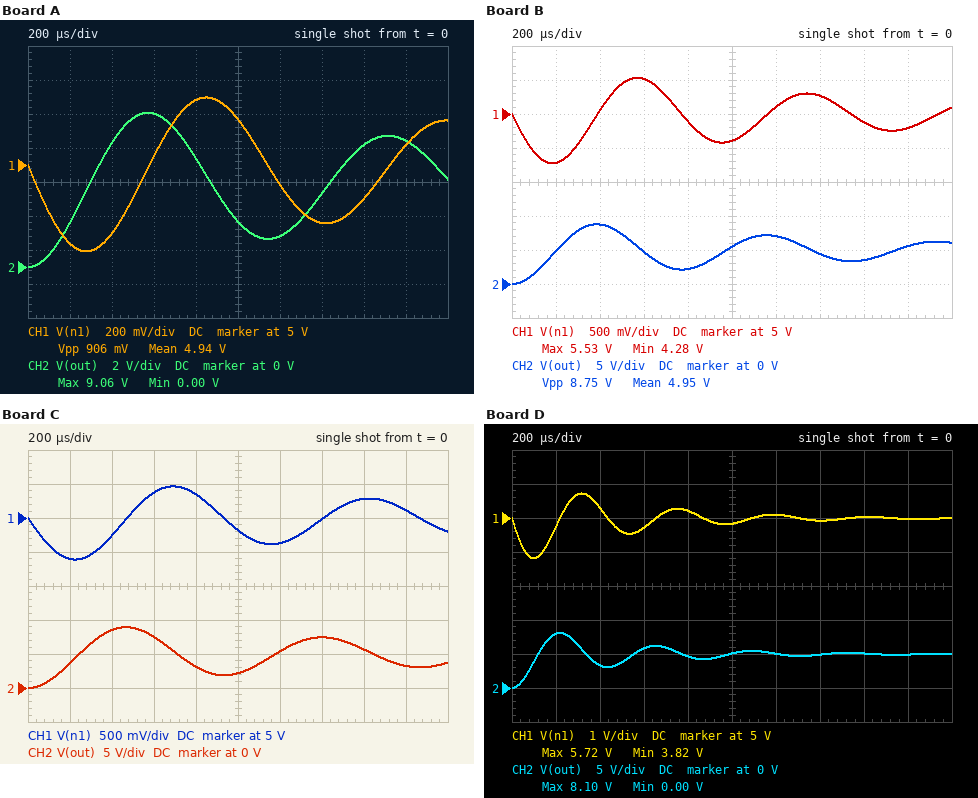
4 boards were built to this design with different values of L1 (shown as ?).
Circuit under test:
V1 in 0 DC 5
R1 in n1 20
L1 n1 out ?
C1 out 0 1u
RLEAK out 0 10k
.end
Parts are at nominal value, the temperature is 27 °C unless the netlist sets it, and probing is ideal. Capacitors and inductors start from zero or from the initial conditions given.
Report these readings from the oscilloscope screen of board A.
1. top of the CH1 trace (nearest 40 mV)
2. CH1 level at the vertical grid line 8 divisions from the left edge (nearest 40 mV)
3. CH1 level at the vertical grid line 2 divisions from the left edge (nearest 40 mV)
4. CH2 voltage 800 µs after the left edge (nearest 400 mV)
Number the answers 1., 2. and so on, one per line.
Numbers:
1. 5.40 V
2. 4.80 V
3. 4.60 V
4. 6.4 V
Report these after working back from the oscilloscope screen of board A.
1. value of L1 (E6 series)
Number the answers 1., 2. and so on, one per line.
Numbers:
1. 33 mH
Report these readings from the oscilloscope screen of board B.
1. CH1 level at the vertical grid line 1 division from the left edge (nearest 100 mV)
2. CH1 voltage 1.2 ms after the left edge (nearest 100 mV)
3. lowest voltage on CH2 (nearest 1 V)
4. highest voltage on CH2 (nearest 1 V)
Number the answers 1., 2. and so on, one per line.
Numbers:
1. 4.3 V
2. 5.1 V
3. 0 V
4. 9 V
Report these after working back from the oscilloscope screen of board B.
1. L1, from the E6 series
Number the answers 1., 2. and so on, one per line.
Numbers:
1. 15 mH
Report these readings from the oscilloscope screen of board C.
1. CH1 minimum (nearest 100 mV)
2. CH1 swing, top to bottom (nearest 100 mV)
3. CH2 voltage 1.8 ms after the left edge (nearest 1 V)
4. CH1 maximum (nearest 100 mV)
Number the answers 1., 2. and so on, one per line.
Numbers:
1. 4.4 V
2. 1.1 V
3. 3 V
4. 5.5 V
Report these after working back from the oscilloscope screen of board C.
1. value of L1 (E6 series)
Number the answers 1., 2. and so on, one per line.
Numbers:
1. 22 mH
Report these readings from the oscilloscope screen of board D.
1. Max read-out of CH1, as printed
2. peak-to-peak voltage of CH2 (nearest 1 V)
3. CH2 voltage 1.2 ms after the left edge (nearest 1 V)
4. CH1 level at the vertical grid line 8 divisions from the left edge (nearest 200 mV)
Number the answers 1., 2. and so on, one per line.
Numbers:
1. 5.72 V
2. 8 V
3. 5 V
4. 5.0 V
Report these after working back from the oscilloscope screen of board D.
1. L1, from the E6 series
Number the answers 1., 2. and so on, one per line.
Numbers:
1. 4.7 mH
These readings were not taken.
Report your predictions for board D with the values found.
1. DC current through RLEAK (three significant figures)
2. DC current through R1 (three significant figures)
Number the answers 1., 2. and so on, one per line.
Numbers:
1. 499 µA
2. 499 µA
